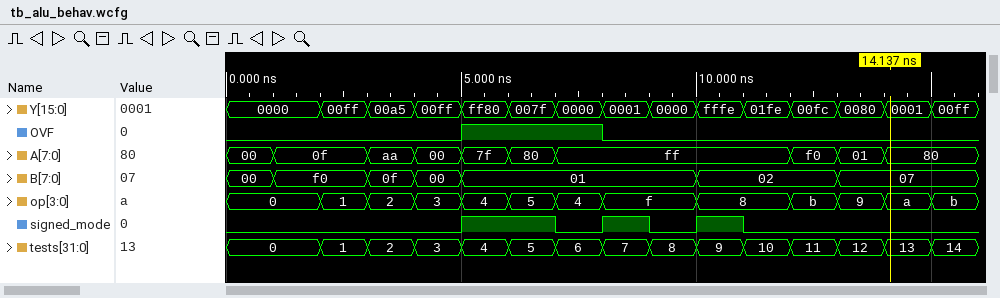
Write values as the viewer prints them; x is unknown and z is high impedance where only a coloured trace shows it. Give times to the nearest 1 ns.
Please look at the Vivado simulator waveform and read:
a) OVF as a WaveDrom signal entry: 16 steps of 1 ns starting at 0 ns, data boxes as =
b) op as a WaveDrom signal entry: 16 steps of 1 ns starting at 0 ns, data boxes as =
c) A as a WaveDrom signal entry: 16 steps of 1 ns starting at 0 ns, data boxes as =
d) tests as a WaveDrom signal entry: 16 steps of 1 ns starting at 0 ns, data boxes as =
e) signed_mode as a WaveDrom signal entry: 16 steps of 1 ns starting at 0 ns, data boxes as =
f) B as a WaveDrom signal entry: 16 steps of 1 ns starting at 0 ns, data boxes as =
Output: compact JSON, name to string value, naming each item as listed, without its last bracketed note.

{"OVF as a WaveDrom signal entry: 16 steps of 1 ns starting at 0 ns, data boxes as =": "{name: 'OVF', wave: '0....1..0.......'}", "op as a WaveDrom signal entry: 16 steps of 1 ns starting at 0 ns, data boxes as =": "{name: 'op', wave: '=.=======.=.====', data: '0 1 2 3 4 5 4 f 8 b 9 a b'}", "A as a WaveDrom signal entry: 16 steps of 1 ns starting at 0 ns, data boxes as =": "{name: 'A', wave: '==.=====....===.', data: '00 0f aa 00 7f 80 ff f0 01 80'}", "tests as a WaveDrom signal entry: 16 steps of 1 ns starting at 0 ns, data boxes as =": "{name: 'tests', wave: '=.==============', data: '0 1 2 3 4 5 6 7 8 9 10 11 12 13 14'}", "signed_mode as a WaveDrom signal entry: 16 steps of 1 ns starting at 0 ns, data boxes as =": "{name: 'signed_mode', wave: '0....1.01010....'}", "B as a WaveDrom signal entry: 16 steps of 1 ns starting at 0 ns, data boxes as =": "{name: 'B', wave: '==.===....=..=..', data: '00 f0 0f 00 01 02 07'}"}
